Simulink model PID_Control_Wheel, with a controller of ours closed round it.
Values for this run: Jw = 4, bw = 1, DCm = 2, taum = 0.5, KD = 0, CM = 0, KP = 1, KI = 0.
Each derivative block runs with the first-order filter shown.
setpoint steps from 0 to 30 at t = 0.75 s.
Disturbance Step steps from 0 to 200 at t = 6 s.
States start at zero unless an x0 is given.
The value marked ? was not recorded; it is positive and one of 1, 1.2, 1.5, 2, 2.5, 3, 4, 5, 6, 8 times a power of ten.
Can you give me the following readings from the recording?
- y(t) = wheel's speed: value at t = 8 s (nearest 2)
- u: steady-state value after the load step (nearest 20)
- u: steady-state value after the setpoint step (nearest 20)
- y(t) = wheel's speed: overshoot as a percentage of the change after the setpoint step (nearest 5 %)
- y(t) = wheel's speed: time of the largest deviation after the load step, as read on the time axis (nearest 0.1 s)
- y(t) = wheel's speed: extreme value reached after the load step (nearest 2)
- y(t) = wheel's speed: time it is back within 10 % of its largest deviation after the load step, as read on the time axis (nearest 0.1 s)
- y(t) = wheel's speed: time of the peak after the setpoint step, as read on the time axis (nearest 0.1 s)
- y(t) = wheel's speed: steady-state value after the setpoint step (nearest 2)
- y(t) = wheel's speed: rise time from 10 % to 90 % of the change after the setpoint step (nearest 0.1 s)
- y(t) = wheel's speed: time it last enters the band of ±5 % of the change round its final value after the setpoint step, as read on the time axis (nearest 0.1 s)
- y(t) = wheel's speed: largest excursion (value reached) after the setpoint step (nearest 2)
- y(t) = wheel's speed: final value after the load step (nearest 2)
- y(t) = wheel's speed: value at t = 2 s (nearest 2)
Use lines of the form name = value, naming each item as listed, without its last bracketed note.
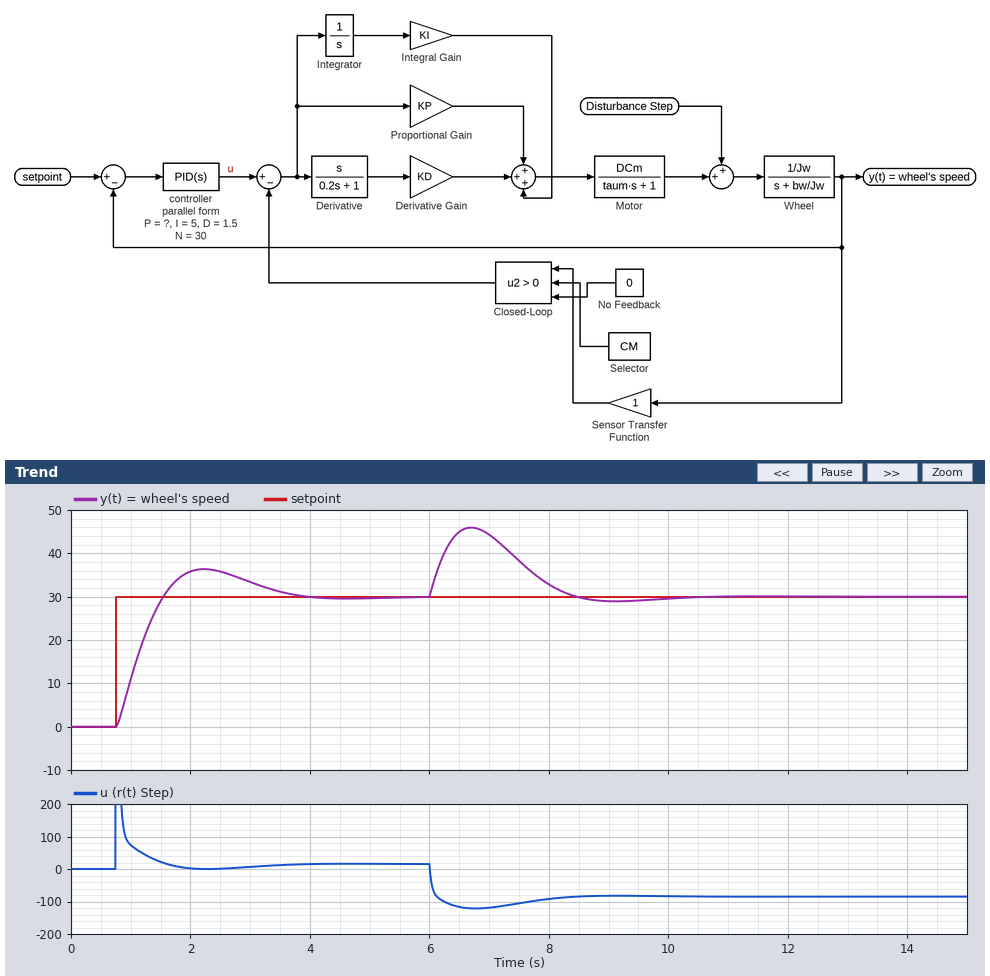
y(t) = wheel's speed: value at t = 8 s = 32
u: steady-state value after the load step = -80
u: steady-state value after the setpoint step = 20
y(t) = wheel's speed: overshoot as a percentage of the change after the setpoint step = 20 %
y(t) = wheel's speed: time of the largest deviation after the load step, as read on the time axis = 6.7 s
y(t) = wheel's speed: extreme value reached after the load step = 46
y(t) = wheel's speed: time it is back within 10 % of its largest deviation after the load step, as read on the time axis = 8.2 s
y(t) = wheel's speed: time of the peak after the setpoint step, as read on the time axis = 2.2 s
y(t) = wheel's speed: steady-state value after the setpoint step = 30
y(t) = wheel's speed: rise time from 10 % to 90 % of the change after the setpoint step = 0.6 s
y(t) = wheel's speed: time it last enters the band of ±5 % of the change round its final value after the setpoint step, as read on the time axis = 3.4 s
y(t) = wheel's speed: largest excursion (value reached) after the setpoint step = 36
y(t) = wheel's speed: final value after the load step = 30
y(t) = wheel's speed: value at t = 2 s = 36
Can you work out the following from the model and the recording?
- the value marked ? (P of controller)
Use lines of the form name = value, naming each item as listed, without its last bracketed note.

the value marked ? = 6
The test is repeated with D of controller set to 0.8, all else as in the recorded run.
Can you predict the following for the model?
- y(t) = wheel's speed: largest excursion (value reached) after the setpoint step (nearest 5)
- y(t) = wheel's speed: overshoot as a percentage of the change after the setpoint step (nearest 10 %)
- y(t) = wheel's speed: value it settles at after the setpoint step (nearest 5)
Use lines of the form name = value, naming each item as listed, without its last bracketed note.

y(t) = wheel's speed: largest excursion (value reached) after the setpoint step = 40
y(t) = wheel's speed: overshoot as a percentage of the change after the setpoint step = 30 %
y(t) = wheel's speed: value it settles at after the setpoint step = 30
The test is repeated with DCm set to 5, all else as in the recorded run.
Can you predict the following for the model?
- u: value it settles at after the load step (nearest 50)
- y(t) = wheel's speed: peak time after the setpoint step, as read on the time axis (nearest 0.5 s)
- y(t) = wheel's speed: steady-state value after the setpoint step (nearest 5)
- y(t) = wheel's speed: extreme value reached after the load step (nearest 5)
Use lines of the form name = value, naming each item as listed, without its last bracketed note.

u: value it settles at after the load step = -50
y(t) = wheel's speed: peak time after the setpoint step, as read on the time axis = 1.5 s
y(t) = wheel's speed: steady-state value after the setpoint step = 30
y(t) = wheel's speed: extreme value reached after the load step = 40
